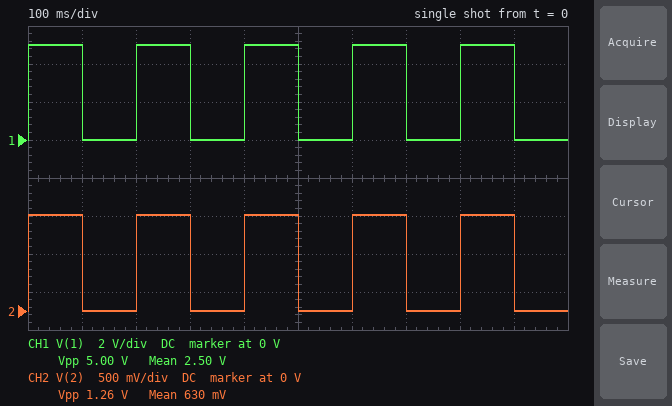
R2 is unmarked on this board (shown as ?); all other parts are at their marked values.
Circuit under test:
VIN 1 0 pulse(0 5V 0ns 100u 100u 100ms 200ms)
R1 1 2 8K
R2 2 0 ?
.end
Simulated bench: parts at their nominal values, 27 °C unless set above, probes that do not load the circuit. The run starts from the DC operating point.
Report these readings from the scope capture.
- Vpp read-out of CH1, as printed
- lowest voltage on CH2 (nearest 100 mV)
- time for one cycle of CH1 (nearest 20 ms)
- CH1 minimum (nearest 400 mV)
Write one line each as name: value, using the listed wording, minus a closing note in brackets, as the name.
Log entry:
Vpp read-out of CH1, as printed: 5.00 V
lowest voltage on CH2: 0 V
time for one cycle of CH1: 200 ms
CH1 minimum: 0 V
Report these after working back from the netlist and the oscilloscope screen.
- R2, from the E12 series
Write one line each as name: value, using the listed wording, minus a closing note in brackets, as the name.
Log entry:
R2, from the E12 series: 2.7 kΩ
